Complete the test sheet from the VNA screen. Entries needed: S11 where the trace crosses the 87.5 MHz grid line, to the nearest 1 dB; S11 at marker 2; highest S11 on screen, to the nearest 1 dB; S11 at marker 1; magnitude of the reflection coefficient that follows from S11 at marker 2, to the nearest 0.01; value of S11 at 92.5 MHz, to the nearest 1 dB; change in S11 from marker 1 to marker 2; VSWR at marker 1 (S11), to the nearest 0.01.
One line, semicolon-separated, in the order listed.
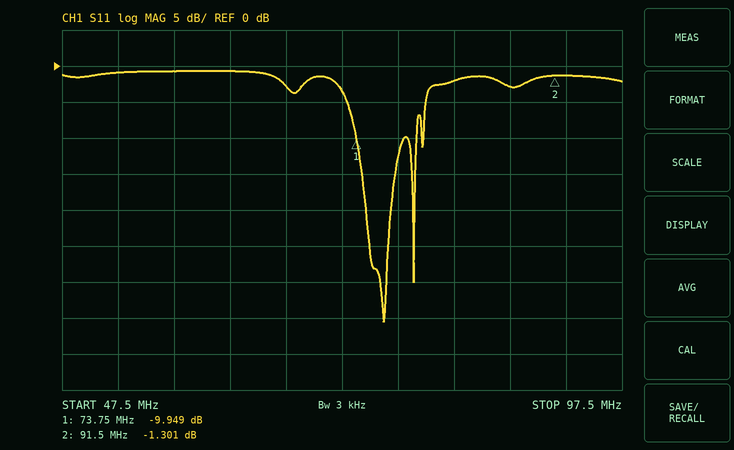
-3 dB; -1.301 dB; -1 dB; -9.949 dB; 0.86; -1 dB; 8.648 dB; 1.93
